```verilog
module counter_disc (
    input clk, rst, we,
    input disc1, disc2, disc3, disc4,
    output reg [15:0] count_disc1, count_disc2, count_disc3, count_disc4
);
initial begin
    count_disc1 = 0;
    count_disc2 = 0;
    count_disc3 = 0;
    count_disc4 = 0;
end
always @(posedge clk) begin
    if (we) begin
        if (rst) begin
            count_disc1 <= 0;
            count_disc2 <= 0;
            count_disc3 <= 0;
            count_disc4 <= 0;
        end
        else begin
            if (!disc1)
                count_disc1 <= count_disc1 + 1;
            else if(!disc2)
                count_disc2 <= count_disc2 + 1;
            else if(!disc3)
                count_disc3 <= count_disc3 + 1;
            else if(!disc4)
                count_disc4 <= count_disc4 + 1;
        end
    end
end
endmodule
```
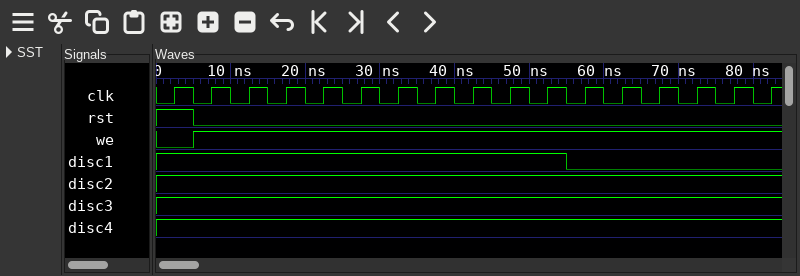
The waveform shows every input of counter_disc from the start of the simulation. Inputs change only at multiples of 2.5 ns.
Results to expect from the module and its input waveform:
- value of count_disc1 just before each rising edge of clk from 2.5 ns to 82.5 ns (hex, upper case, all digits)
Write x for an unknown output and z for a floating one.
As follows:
0000, 0000, 0000, 0000, 0000, 0000, 0000, 0000, 0000, 0000, 0000, 0000, 0001, 0002, 0003, 0004, 0005
